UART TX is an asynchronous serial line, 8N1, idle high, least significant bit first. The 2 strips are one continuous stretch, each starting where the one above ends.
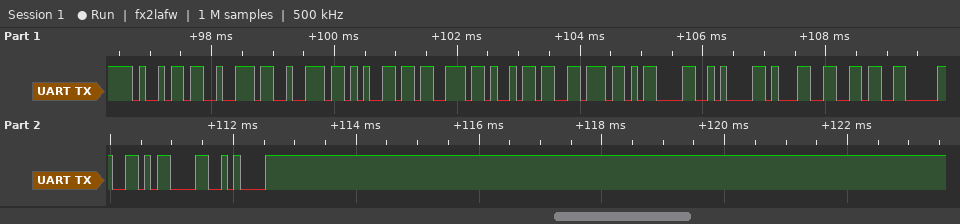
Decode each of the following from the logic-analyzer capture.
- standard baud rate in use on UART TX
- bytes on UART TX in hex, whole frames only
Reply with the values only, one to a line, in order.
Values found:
9600 baud
0x69 0x72 0x72 0x65 0x73 0x69 0x76 0x0D 0x0A 0x31 0x36 0x30 0x0D 0x0A
